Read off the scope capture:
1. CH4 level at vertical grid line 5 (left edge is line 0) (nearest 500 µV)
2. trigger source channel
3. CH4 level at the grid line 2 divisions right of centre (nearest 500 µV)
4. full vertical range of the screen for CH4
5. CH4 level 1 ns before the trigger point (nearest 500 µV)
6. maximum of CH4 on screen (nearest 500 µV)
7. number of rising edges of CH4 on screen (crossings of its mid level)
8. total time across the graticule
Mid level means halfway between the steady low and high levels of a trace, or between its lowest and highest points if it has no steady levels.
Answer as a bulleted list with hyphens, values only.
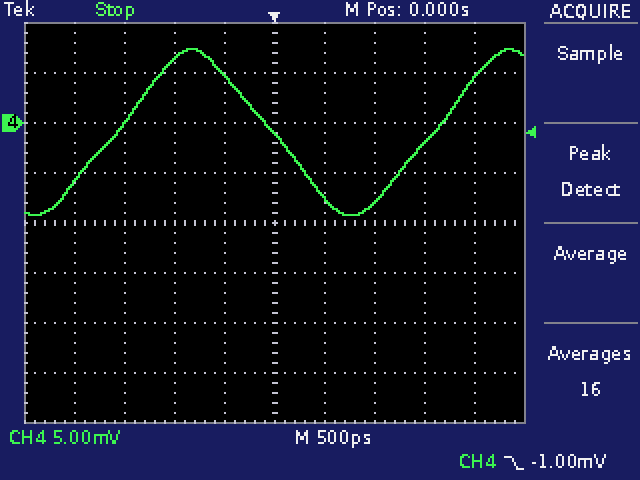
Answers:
- -1.0 mV
- CH4
- -8.0 mV
- 40 mV
- 6.5 mV
- 7.5 mV
- 2
- 5 ns
